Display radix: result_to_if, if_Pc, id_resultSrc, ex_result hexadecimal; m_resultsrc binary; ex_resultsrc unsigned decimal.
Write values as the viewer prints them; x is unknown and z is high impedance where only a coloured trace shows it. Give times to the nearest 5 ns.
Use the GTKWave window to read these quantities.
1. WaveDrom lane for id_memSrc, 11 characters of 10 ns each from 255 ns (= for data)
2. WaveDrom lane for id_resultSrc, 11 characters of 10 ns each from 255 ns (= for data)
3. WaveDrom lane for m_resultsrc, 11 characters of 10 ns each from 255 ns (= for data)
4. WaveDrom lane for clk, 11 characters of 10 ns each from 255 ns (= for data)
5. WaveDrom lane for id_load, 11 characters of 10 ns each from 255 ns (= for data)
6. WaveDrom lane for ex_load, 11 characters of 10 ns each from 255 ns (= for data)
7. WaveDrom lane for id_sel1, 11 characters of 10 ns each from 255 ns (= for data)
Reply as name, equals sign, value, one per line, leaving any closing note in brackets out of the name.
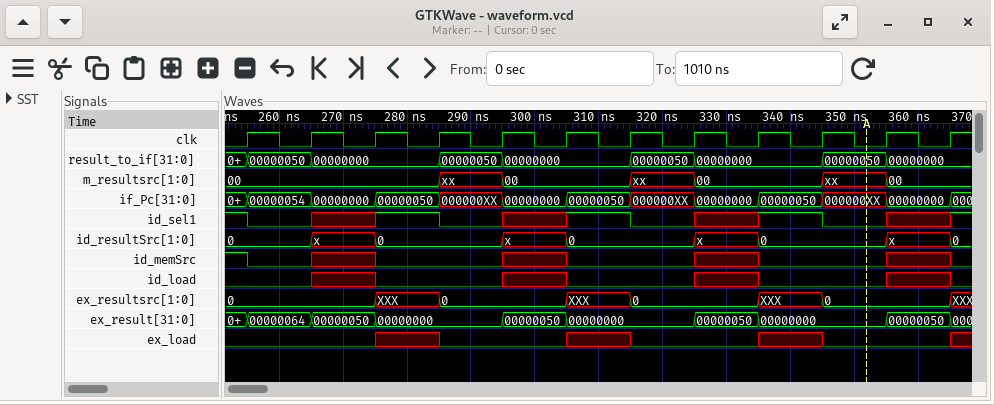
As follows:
WaveDrom lane for id_memSrc, 11 characters of 10 ns each from 255 ns = {name: 'id_memSrc', wave: '0x0.x0.x0.x'}
WaveDrom lane for id_resultSrc, 11 characters of 10 ns each from 255 ns = {name: 'id_resultSrc', wave: '=x=.x=.x=.x', data: '0 0 0 0'}
WaveDrom lane for m_resultsrc, 11 characters of 10 ns each from 255 ns = {name: 'm_resultsrc', wave: '=..x=.x=.x=', data: '00 00 00 00'}
WaveDrom lane for clk, 11 characters of 10 ns each from 255 ns = {name: 'clk', wave: 'p..........'}
WaveDrom lane for id_load, 11 characters of 10 ns each from 255 ns = {name: 'id_load', wave: '0x0.x0.x0.x'}
WaveDrom lane for ex_load, 11 characters of 10 ns each from 255 ns = {name: 'ex_load', wave: '0.x0.x0.x0.'}
WaveDrom lane for id_sel1, 11 characters of 10 ns each from 255 ns = {name: 'id_sel1', wave: '0x10x10x10x'}
